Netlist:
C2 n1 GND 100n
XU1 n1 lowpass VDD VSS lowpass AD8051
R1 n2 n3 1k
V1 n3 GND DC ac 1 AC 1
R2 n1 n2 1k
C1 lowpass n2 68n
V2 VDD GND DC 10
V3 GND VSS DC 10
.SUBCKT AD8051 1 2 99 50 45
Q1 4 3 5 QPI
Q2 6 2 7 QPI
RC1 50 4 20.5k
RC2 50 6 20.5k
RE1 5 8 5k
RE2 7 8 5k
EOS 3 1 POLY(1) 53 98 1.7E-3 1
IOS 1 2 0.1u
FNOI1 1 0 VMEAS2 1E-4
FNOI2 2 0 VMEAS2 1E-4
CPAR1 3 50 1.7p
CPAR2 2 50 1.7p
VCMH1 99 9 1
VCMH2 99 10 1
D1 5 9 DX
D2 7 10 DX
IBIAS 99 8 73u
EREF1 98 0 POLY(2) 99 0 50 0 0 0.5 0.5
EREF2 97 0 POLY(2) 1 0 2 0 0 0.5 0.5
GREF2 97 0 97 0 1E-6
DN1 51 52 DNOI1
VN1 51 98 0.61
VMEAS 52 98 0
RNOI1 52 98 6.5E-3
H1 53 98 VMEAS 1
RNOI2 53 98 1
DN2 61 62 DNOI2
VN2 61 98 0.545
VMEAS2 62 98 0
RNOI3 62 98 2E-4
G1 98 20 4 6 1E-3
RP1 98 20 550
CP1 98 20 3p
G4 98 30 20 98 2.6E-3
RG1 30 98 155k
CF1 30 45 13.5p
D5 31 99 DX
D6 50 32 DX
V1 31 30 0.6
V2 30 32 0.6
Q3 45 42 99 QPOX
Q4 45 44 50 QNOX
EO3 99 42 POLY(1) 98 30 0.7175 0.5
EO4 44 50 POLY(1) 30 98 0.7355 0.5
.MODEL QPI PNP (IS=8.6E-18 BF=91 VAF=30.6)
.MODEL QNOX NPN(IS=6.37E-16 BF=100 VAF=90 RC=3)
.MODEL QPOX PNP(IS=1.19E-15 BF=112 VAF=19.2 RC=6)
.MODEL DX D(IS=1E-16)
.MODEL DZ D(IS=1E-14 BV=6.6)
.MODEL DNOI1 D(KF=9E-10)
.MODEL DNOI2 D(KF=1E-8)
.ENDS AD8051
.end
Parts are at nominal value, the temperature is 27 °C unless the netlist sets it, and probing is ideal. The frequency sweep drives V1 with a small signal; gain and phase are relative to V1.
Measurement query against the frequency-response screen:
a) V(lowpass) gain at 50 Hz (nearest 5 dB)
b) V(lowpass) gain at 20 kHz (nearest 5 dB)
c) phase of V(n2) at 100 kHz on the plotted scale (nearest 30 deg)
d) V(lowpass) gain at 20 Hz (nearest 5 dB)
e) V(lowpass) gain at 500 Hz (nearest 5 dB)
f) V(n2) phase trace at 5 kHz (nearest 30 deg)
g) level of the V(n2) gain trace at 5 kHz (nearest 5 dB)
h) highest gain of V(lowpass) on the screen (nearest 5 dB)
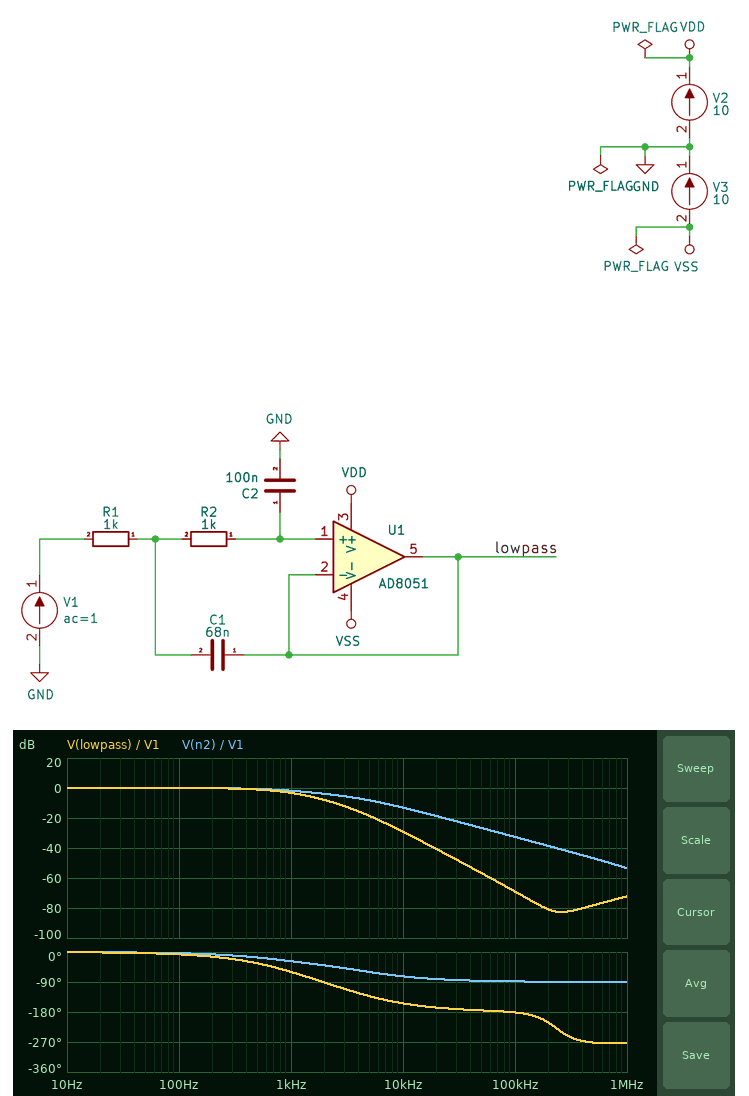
0 dB
-40 dB
-90 deg
0 dB
0 dB
-60 deg
-10 dB
0 dB
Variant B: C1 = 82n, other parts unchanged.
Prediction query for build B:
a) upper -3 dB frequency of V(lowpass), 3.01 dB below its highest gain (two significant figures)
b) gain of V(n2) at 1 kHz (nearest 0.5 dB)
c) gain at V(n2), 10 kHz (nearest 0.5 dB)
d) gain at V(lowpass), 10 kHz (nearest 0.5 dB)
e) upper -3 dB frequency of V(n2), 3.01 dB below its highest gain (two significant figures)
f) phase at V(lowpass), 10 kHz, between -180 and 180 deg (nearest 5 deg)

980 Hz
-1.5 dB
-14.5 dB
-30.5 dB
1.6 kHz
-160 deg
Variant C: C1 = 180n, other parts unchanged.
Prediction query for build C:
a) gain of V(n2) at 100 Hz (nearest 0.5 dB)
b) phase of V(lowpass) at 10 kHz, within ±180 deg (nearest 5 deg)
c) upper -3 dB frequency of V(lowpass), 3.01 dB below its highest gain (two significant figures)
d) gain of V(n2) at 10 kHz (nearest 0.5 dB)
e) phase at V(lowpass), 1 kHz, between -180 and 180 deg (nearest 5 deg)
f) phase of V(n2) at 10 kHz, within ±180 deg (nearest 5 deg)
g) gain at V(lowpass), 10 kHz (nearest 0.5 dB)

0 dB
-170 deg
1.1 kHz
-21.0 dB
-75 deg
-90 deg
-37.0 dB
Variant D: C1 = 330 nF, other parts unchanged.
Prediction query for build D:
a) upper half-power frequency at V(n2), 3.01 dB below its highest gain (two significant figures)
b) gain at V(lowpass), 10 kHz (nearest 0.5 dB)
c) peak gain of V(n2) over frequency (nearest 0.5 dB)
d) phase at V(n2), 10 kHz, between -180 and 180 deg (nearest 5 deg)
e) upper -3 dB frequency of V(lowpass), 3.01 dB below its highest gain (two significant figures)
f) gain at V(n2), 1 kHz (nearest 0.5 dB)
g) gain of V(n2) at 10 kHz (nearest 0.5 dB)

1.1 kHz
-42.5 dB
1.5 dB
-95 deg
1.0 kHz
-1.0 dB
-26.0 dB
